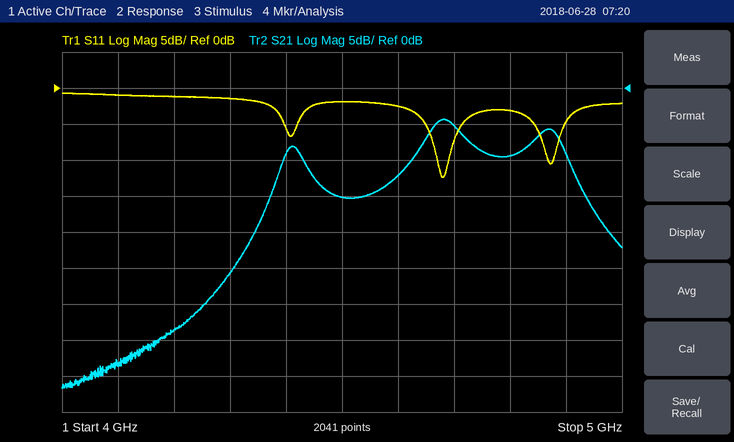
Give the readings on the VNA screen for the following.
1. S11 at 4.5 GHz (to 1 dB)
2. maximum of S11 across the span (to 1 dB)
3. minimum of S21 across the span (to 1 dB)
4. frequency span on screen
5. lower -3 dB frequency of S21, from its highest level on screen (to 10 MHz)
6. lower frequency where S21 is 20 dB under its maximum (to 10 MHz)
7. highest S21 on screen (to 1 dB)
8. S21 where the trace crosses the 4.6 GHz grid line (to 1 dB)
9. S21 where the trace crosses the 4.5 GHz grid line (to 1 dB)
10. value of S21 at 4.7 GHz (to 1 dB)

-2 dB
-1 dB
-42 dB
1 GHz
4.65 GHz
4.31 GHz
-4 dB
-12 dB
-15 dB
-5 dB
